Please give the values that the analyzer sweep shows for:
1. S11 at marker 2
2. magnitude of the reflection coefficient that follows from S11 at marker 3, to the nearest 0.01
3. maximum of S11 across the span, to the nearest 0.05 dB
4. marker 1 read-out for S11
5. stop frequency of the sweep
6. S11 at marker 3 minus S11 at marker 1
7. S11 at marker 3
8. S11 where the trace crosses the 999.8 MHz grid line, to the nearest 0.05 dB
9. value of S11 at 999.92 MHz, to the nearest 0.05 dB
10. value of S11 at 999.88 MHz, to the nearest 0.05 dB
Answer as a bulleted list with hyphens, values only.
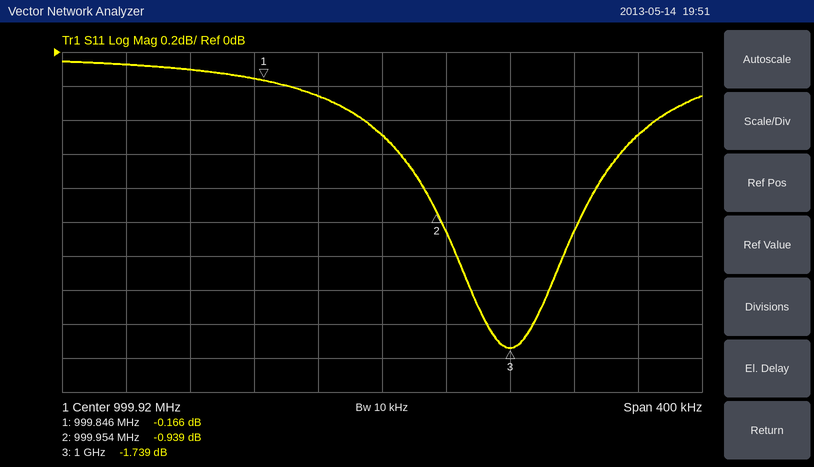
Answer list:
- -0.939 dB
- 0.82
- -0.05 dB
- -0.166 dB
- 1.00012 GHz
- -1.573 dB
- -1.739 dB
- -0.10 dB
- -0.50 dB
- -0.25 dB
